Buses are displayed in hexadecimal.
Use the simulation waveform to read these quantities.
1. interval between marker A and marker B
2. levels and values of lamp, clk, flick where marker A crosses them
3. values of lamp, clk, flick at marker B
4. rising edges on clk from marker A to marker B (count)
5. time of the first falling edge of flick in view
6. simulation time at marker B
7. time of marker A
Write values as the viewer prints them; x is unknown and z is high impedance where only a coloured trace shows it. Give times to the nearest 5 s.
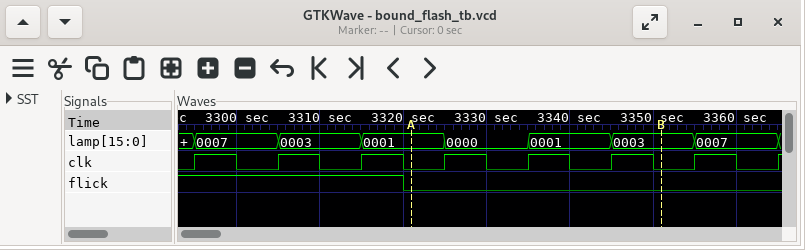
30 s
lamp=0001, clk=0, flick=0
lamp=0003, clk=0, flick=0
3
3320 s
3350 s
3320 s
